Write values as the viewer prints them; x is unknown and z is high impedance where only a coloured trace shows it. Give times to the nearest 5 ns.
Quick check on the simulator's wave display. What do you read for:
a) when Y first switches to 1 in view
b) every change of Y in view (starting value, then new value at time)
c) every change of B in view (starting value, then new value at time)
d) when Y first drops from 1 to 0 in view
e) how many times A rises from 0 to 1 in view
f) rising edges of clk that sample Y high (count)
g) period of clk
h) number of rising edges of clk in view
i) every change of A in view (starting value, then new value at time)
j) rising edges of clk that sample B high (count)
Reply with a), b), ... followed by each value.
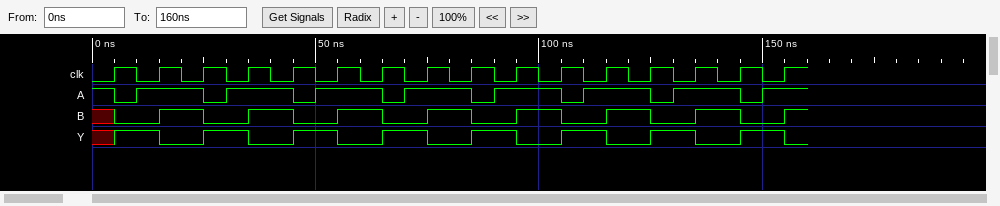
a) 5 ns
b) x, 1 at 5 ns, 0 at 15 ns, 1 at 25 ns, 0 at 35 ns, 1 at 45 ns, 0 at 55 ns, 1 at 65 ns, 0 at 75 ns, 1 at 85 ns, 0 at 95 ns, 1 at 105 ns, 0 at 115 ns, 1 at 125 ns, 0 at 135 ns, 1 at 145 ns, 0 at 155 ns
c) x, 0 at 5 ns, 1 at 15 ns, 0 at 25 ns, 1 at 35 ns, 0 at 45 ns, 1 at 55 ns, 0 at 65 ns, 1 at 75 ns, 0 at 85 ns, 1 at 95 ns, 0 at 105 ns, 1 at 115 ns, 0 at 125 ns, 1 at 135 ns, 0 at 145 ns, 1 at 155 ns
d) 15 ns
e) 8
f) 8
g) 10 ns
h) 16
i) 1, 0 at 5 ns, 1 at 10 ns, 0 at 25 ns, 1 at 30 ns, 0 at 45 ns, 1 at 50 ns, 0 at 65 ns, 1 at 70 ns, 0 at 85 ns, 1 at 90 ns, 0 at 105 ns, 1 at 110 ns, 0 at 125 ns, 1 at 130 ns, 0 at 145 ns, 1 at 150 ns
j) 7
